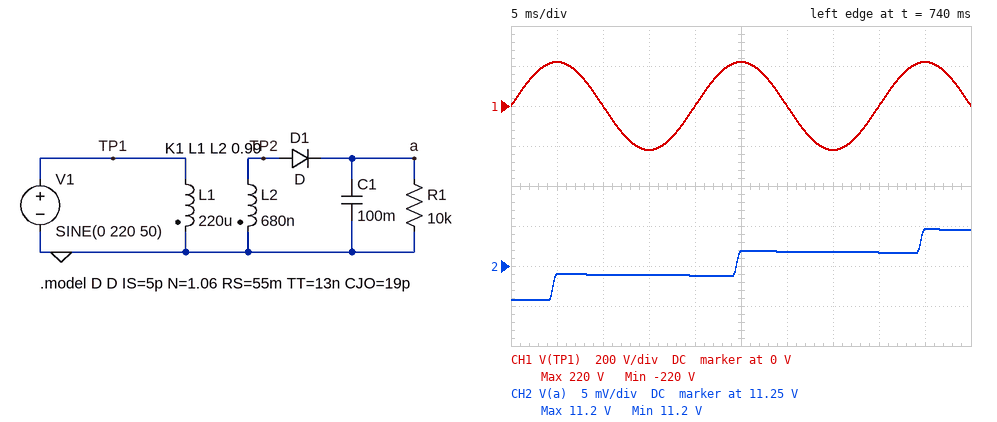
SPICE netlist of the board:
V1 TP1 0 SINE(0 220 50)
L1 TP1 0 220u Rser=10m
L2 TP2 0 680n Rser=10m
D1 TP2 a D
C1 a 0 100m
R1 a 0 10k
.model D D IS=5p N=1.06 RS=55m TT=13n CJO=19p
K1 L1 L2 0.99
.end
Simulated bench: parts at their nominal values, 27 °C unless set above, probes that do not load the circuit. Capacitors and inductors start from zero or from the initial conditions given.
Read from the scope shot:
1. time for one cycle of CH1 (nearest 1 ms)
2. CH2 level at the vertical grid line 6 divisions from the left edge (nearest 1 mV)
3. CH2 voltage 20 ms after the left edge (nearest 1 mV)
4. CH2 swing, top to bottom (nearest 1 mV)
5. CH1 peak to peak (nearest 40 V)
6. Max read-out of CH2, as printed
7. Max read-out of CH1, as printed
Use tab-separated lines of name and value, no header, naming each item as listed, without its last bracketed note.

time for one cycle of CH1	20 ms
CH2 level at the vertical grid line 6 divisions from the left edge	11.247 V
CH2 voltage 20 ms after the left edge	11.244 V
CH2 swing, top to bottom	9 mV
CH1 peak to peak	440 V
Max read-out of CH2, as printed	11.2 V
Max read-out of CH1, as printed	220 V
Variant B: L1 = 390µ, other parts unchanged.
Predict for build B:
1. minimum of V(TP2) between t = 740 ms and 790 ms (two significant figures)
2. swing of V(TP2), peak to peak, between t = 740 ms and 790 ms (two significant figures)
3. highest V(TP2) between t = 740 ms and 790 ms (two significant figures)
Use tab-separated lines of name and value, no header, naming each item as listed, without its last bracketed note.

minimum of V(TP2) between t = 740 ms and 790 ms	-9.1 V
swing of V(TP2), peak to peak, between t = 740 ms and 790 ms	18 V
highest V(TP2) between t = 740 ms and 790 ms	9.1 V
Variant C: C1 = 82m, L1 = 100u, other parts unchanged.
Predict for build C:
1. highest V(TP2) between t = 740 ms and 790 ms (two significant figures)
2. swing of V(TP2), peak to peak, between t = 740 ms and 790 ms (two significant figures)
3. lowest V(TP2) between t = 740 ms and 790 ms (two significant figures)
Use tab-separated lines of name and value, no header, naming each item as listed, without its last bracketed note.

highest V(TP2) between t = 740 ms and 790 ms	17 V
swing of V(TP2), peak to peak, between t = 740 ms and 790 ms	34 V
lowest V(TP2) between t = 740 ms and 790 ms	-17 V
